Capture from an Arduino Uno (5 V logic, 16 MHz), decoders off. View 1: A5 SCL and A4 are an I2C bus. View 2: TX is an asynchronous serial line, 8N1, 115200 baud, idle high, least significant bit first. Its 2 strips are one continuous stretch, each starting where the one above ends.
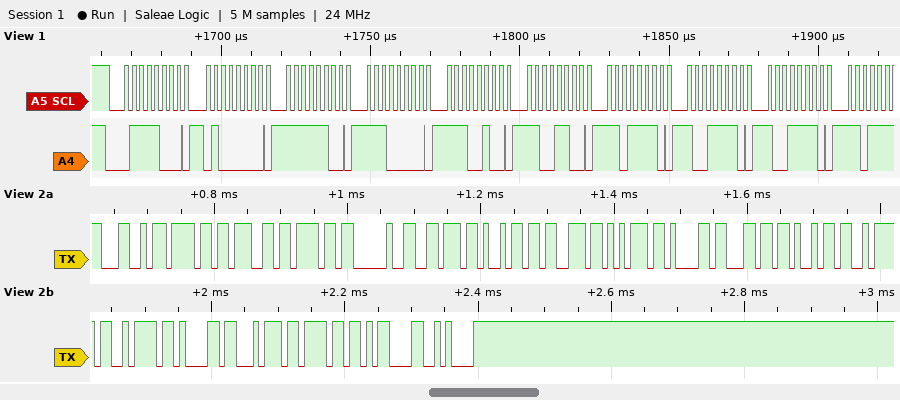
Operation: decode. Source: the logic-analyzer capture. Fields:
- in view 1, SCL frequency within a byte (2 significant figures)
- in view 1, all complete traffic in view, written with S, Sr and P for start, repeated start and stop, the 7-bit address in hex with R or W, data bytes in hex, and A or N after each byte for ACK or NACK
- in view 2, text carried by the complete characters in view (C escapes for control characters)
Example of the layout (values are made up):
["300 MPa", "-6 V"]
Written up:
["400 kHz", "S 3CW A 40 A FC A E0 A E4 A CC A DE A 9E A 9E A", "\"Logo visualizzato\\r\\n\""]
